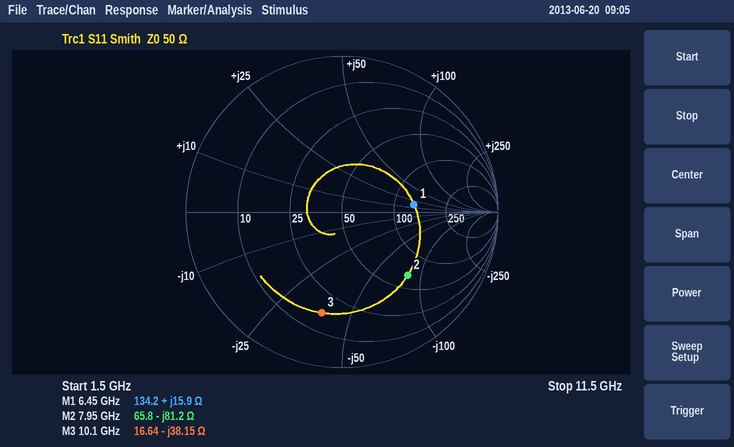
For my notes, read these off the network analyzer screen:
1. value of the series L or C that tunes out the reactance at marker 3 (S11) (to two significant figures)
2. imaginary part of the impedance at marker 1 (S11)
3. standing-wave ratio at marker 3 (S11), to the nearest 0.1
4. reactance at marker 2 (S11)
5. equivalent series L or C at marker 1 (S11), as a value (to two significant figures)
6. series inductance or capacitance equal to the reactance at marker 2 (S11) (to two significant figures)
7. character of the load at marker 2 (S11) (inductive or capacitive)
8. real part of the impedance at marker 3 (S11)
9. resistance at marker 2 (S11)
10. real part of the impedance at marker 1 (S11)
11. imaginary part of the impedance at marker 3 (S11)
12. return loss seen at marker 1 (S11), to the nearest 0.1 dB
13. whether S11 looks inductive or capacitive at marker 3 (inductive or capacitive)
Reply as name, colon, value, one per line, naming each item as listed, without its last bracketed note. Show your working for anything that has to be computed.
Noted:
value of the series L or C that tunes out the reactance at marker 3 (S11): L = 38.15 Ω/(2π × 10.1 GHz) ≈ 601 pH, so 600 pH to two significant figures
imaginary part of the impedance at marker 1: +15.9 Ω
standing-wave ratio at marker 3 (S11), to the nearest 0.1: 4.9
reactance at marker 2: -81.2 Ω
equivalent series L or C at marker 1 (S11), as a value: L = 15.9 Ω/(2π × 6.45 GHz) ≈ 392 pH, so 390 pH to two significant figures
series inductance or capacitance equal to the reactance at marker 2 (S11): C = 1/(2π × 7.95 GHz × 81.2 Ω) ≈ 247 fF, so 250 fF to two significant figures
character of the load at marker 2 (S11): capacitive
real part of the impedance at marker 3: 16.64 Ω
resistance at marker 2: 65.8 Ω
real part of the impedance at marker 1: 134.2 Ω
imaginary part of the impedance at marker 3: -38.15 Ω
return loss seen at marker 1 (S11), to the nearest 0.1 dB: 6.7 dB
whether S11 looks inductive or capacitive at marker 3: capacitive
